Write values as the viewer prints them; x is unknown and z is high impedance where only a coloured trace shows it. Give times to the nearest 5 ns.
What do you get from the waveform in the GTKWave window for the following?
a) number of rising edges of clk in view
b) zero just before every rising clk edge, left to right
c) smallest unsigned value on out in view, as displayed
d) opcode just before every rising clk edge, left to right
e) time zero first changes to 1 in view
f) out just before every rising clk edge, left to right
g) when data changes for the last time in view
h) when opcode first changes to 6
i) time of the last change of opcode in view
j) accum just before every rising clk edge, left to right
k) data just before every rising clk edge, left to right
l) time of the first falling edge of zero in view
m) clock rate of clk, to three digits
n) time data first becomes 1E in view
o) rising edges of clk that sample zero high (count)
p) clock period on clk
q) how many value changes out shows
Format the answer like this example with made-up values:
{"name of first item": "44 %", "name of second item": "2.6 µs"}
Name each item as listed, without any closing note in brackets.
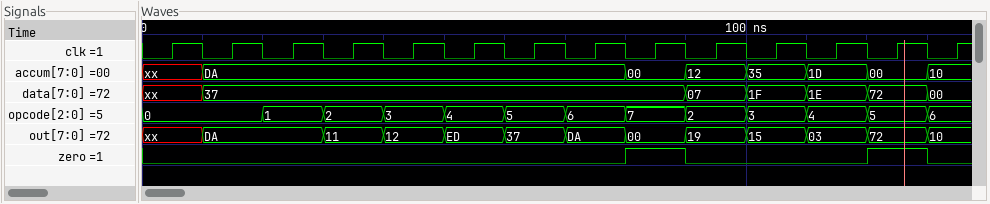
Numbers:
{"number of rising edges of clk in view": "14", "zero just before every rising clk edge, left to right": "0 0 0 0 0 0 0 0 1 0 0 0 1 0", "smallest unsigned value on out in view, as displayed": "00", "opcode just before every rising clk edge, left to right": "0, 0, 1, 2, 3, 4, 5, 6, 7, 2, 3, 4, 5, 6", "time zero first changes to 1 in view": "80 ns", "out just before every rising clk edge, left to right": "xx, DA, DA, 11, 12, ED, 37, DA, 00, 19, 15, 03, 72, 10", "when data changes for the last time in view": "130 ns", "when opcode first changes to 6": "70 ns", "time of the last change of opcode in view": "130 ns", "accum just before every rising clk edge, left to right": "xx, DA, DA, DA, DA, DA, DA, DA, 00, 12, 35, 1D, 00, 10", "data just before every rising clk edge, left to right": "xx, 37, 37, 37, 37, 37, 37, 37, 37, 07, 1F, 1E, 72, 00", "time of the first falling edge of zero in view": "90 ns", "clock rate of clk, to three digits": "100 MHz", "time data first becomes 1E in view": "110 ns", "rising edges of clk that sample zero high": "2", "clock period on clk": "10 ns", "how many value changes out shows": "12"}
